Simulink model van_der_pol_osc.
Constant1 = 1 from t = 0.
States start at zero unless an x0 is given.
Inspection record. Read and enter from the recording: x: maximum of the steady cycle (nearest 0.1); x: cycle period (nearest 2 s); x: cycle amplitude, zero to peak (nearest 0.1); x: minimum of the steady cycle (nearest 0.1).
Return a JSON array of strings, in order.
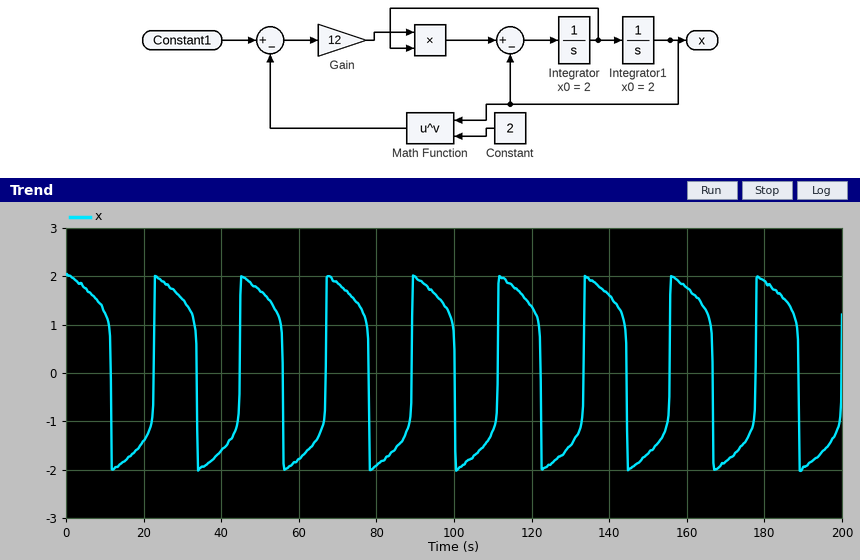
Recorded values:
["2.0", "22 s", "2.0", "-2.0"]
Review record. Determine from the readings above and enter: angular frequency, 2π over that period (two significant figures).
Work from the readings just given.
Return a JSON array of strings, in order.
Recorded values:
["0.29 rad/s"]
